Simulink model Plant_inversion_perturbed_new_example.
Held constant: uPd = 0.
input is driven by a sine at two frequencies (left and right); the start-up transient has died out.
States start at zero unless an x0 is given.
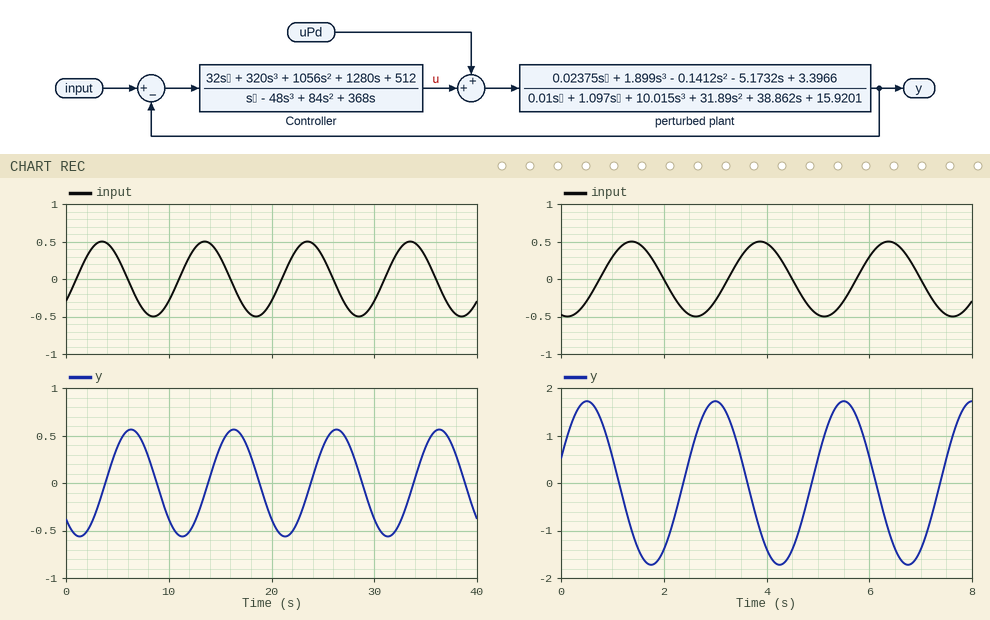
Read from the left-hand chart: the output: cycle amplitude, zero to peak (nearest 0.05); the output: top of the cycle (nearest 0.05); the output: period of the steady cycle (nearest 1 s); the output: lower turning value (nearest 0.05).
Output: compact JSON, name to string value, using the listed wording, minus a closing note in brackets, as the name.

{"the output: cycle amplitude, zero to peak": "0.55", "the output: top of the cycle": "0.55", "the output: period of the steady cycle": "10 s", "the output: lower turning value": "-0.55"}
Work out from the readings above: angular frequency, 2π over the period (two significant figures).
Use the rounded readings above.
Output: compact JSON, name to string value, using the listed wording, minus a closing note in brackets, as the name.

{"angular frequency, 2π over the period": "0.63 rad/s"}
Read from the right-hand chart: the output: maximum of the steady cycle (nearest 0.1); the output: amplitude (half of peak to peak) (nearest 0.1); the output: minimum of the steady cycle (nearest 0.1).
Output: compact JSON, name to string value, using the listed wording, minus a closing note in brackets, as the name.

{"the output: maximum of the steady cycle": "1.7", "the output: amplitude (half of peak to peak)": "1.7", "the output: minimum of the steady cycle": "-1.7"}
